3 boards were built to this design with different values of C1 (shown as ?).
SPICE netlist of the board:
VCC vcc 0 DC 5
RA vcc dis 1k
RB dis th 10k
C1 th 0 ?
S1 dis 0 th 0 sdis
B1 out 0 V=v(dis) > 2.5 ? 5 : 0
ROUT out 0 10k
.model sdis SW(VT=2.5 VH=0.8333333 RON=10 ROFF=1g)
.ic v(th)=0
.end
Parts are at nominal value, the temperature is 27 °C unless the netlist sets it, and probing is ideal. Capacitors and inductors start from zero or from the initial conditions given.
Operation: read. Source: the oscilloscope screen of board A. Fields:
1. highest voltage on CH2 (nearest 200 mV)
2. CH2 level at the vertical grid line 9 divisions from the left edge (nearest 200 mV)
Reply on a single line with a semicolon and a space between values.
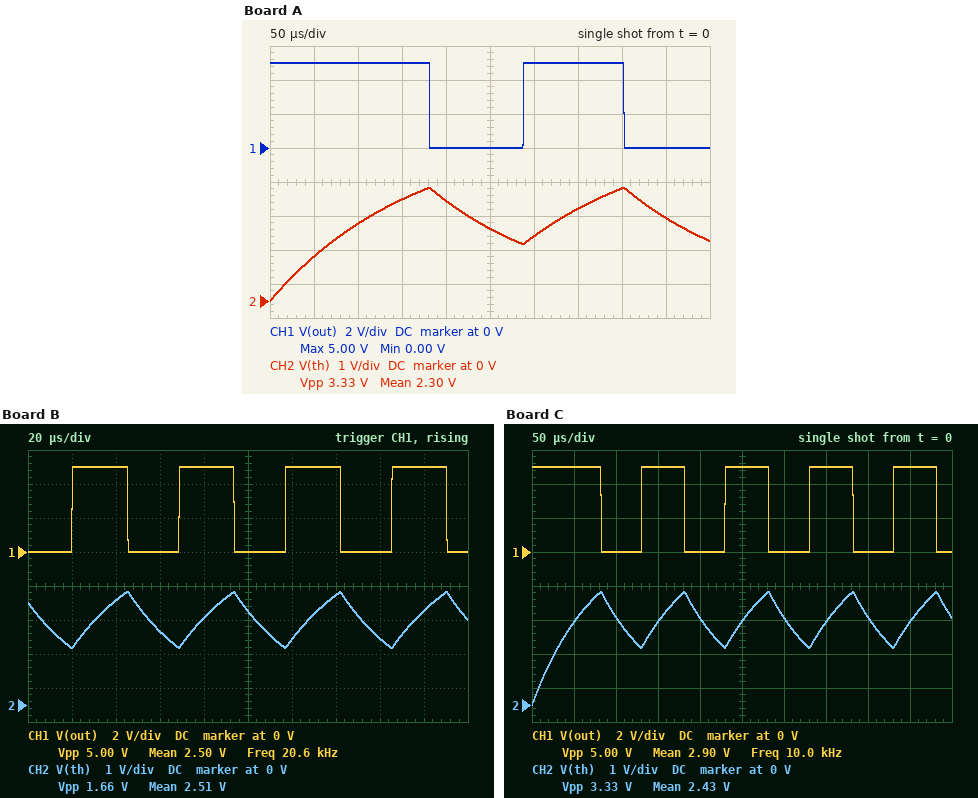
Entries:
3.4 V; 2.4 V
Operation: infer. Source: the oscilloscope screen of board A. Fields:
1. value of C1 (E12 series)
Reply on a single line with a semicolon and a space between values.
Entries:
15 nF
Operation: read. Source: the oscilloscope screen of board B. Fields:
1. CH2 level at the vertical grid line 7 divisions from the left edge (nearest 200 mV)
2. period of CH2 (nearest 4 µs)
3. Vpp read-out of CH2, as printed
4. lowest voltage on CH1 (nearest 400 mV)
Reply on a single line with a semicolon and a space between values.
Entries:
3.2 V; 48 µs; 1.66 V; 0 V
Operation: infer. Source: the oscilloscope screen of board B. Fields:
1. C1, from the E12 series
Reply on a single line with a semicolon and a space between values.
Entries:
3.3 nF
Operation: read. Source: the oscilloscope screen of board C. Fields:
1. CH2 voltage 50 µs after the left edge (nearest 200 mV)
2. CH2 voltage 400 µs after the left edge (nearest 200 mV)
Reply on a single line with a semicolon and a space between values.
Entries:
2.4 V; 2.6 V
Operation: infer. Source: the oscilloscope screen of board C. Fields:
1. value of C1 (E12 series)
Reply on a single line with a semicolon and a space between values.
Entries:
6.8 nF
